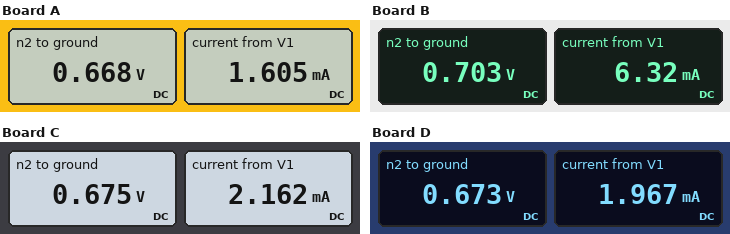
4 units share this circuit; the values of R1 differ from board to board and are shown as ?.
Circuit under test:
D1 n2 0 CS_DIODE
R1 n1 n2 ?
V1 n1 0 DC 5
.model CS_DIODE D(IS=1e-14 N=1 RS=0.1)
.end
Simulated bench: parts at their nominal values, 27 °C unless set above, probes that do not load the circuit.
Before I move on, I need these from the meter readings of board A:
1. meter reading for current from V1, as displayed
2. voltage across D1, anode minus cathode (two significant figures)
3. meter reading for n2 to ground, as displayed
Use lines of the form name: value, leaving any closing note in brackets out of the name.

meter reading for current from V1, as displayed: 1.605 mA
voltage across D1, anode minus cathode: 670 mV
meter reading for n2 to ground, as displayed: 0.668 V
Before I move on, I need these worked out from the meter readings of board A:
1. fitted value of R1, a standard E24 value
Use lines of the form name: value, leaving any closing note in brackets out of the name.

fitted value of R1, a standard E24 value: 2.7 kΩ
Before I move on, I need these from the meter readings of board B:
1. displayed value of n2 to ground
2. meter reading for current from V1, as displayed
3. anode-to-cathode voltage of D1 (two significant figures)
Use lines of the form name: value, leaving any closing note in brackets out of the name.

displayed value of n2 to ground: 0.703 V
meter reading for current from V1, as displayed: 6.32 mA
anode-to-cathode voltage of D1: 700 mV
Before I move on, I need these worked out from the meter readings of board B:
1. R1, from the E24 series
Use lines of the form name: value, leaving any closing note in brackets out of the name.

R1, from the E24 series: 680 Ω
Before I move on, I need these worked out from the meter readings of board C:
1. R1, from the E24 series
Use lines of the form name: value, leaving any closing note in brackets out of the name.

R1, from the E24 series: 2 kΩ
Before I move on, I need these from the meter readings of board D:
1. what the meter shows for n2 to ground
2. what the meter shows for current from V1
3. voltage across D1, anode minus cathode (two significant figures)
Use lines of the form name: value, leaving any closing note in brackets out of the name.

what the meter shows for n2 to ground: 0.673 V
what the meter shows for current from V1: 1.967 mA
voltage across D1, anode minus cathode: 670 mV
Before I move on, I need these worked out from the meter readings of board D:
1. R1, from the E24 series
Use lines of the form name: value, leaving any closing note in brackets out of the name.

R1, from the E24 series: 2.2 kΩ
